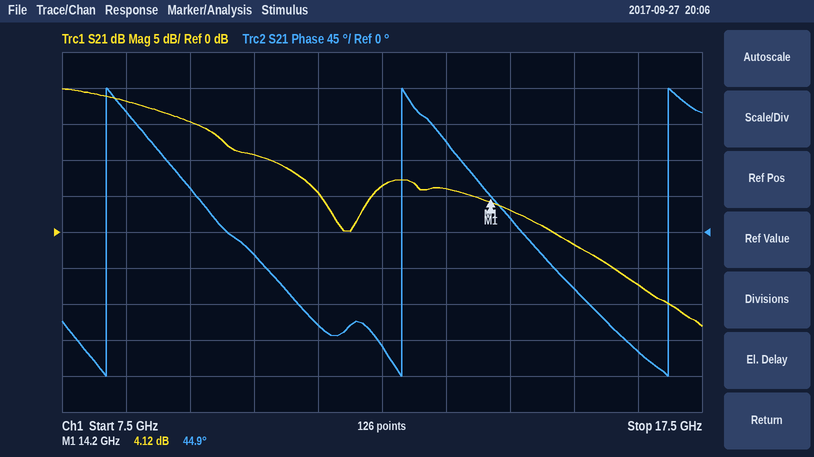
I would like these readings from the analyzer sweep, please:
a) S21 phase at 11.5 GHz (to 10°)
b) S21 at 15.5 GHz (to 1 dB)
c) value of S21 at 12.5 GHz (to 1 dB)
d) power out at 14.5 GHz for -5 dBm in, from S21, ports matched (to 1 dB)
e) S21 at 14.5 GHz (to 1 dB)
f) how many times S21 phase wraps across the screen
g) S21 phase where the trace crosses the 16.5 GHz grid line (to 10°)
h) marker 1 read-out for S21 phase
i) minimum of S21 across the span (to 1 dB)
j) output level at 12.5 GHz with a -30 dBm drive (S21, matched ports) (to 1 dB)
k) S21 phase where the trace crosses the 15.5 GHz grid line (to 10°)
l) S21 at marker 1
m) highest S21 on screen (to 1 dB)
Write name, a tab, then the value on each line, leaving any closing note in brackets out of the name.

S21 phase at 11.5 GHz	-120°
S21 at 15.5 GHz	-2 dB
value of S21 at 12.5 GHz	6 dB
power out at 14.5 GHz for -5 dBm in, from S21, ports matched	-2 dBm
S21 at 14.5 GHz	3 dB
how many times S21 phase wraps across the screen	3
S21 phase where the trace crosses the 16.5 GHz grid line	-150°
marker 1 read-out for S21 phase	44.9°
minimum of S21 across the span	-13 dB
output level at 12.5 GHz with a -30 dBm drive (S21, matched ports)	-24 dBm
S21 phase where the trace crosses the 15.5 GHz grid line	-70°
S21 at marker 1	4.12 dB
highest S21 on screen	20 dB
